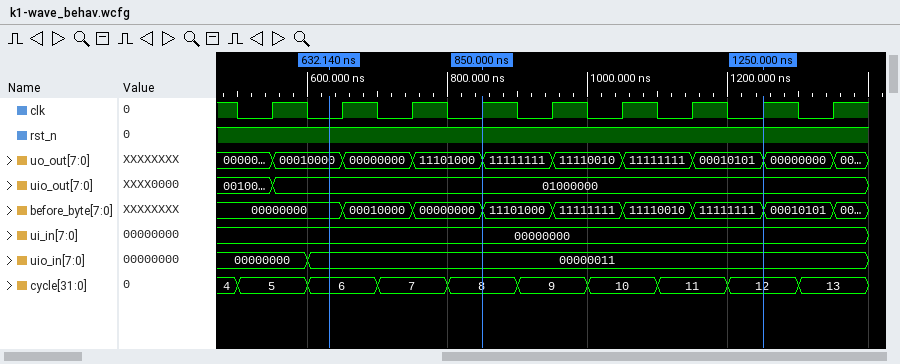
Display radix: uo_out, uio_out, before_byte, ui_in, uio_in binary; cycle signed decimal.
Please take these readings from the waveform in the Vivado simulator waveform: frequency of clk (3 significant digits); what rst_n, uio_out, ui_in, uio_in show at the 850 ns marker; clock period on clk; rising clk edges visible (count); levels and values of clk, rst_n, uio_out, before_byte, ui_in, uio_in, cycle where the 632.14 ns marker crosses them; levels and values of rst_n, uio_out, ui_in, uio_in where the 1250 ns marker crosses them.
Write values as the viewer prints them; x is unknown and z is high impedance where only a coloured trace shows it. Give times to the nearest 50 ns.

10.0 MHz
rst_n=1, uio_out=01000000, ui_in=00000000, uio_in=00000011
100 ns
9
clk=0, rst_n=1, uio_out=01000000, before_byte=00000000, ui_in=00000000, uio_in=00000011, cycle=6
rst_n=1, uio_out=01000000, ui_in=00000000, uio_in=00000011
